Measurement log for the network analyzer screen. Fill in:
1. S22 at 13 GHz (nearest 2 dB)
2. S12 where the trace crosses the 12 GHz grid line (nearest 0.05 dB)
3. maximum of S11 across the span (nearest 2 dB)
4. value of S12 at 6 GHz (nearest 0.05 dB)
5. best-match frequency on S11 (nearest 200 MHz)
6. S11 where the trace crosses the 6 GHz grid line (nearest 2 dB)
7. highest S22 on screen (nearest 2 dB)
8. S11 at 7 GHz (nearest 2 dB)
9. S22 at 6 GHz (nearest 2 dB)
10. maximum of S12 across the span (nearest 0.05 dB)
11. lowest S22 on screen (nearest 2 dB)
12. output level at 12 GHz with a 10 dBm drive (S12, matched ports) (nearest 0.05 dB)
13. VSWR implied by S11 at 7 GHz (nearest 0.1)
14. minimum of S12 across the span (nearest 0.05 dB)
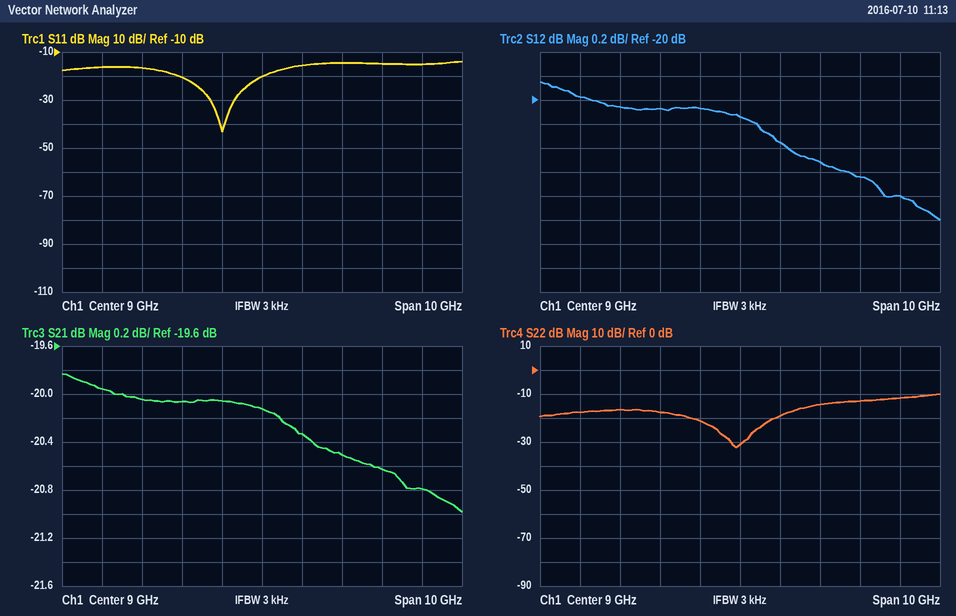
-12 dB
-20.65 dB
-14 dB
-20.05 dB
8.0 GHz
-16 dB
-10 dB
-20 dB
-16 dB
-19.85 dB
-32 dB
-10.65 dBm
1.2
-21.00 dB
